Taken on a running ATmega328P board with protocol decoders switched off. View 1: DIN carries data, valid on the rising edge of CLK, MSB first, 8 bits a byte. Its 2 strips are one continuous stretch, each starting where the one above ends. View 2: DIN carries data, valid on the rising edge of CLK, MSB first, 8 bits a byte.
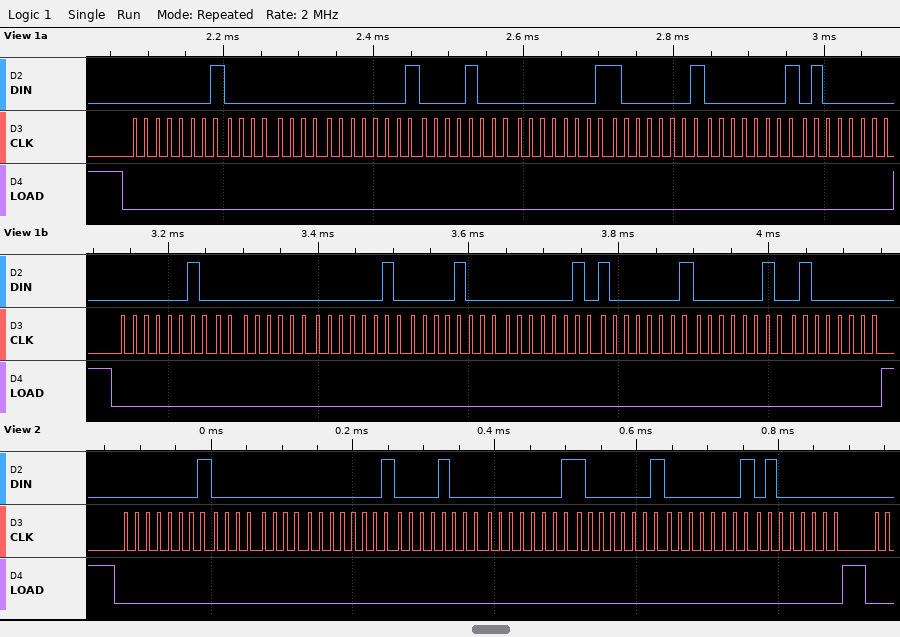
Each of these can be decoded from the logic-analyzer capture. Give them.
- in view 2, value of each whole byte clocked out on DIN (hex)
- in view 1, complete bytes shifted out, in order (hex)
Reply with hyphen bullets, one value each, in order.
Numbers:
- 01 00 01 08 01 81 01 40
- 01 00 01 08 01 81 01 40 02 00 02 08 02 81 02 40
